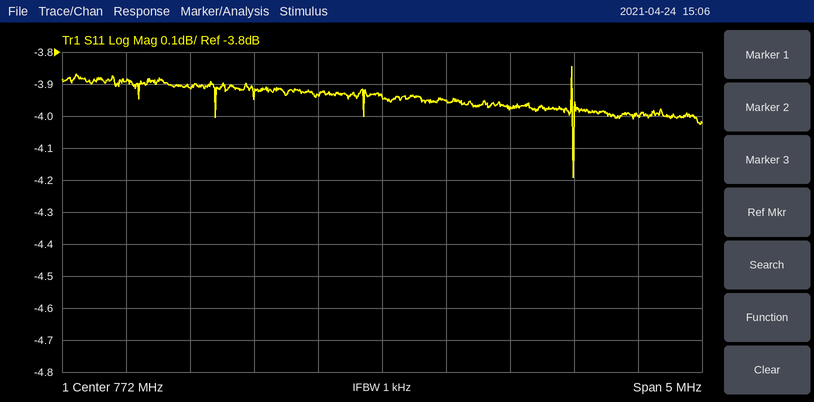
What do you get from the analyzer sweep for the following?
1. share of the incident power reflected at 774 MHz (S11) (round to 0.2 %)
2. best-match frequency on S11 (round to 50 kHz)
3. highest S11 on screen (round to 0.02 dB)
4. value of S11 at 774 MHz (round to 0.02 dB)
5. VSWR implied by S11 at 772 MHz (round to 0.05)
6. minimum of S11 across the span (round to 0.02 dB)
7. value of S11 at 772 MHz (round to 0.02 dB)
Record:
39.8 %
773.50 MHz
-3.84 dB
-4.00 dB
4.50
-4.20 dB
-3.94 dB
